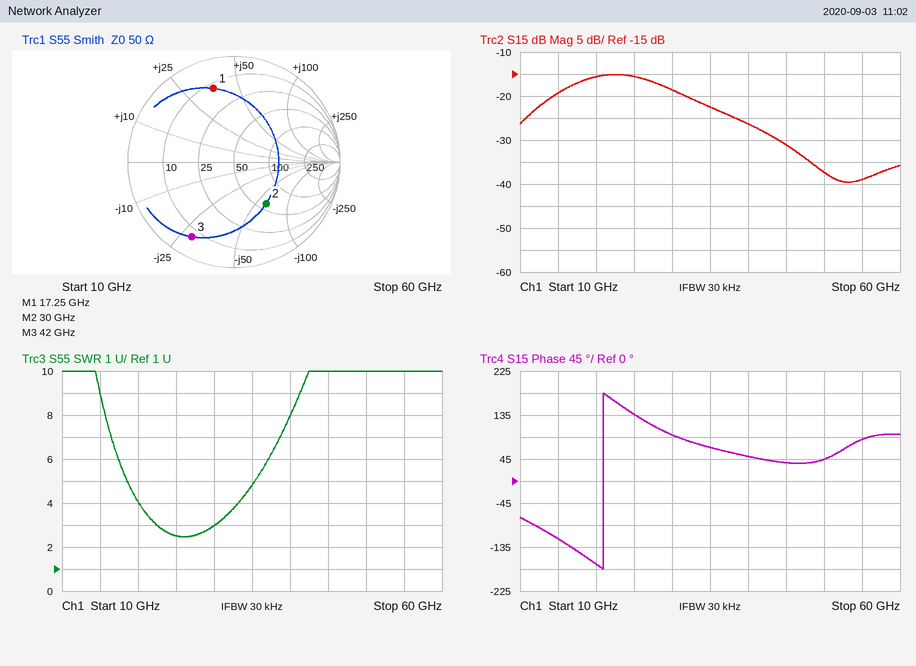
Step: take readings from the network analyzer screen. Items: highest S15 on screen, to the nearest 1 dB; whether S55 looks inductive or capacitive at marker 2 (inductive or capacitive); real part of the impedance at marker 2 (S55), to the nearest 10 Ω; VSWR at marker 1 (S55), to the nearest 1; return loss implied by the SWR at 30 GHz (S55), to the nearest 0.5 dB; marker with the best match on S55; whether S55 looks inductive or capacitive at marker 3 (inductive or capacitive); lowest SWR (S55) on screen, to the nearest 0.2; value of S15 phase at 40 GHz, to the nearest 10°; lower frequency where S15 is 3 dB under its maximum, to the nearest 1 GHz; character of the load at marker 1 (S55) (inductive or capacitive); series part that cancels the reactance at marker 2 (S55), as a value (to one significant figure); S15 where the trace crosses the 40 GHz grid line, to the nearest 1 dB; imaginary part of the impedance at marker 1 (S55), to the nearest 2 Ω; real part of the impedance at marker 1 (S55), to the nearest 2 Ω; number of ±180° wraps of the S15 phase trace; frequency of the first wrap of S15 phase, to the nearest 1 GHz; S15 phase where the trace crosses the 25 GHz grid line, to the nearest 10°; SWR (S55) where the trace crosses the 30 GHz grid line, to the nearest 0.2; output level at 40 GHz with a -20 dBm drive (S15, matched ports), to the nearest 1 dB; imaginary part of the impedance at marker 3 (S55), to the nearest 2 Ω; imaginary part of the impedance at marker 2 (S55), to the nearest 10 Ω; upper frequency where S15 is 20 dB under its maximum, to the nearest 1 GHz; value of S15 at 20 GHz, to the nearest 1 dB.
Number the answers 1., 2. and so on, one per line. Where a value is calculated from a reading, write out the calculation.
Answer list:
1. -15 dB
2. capacitive
3. 60 Ω
4. 6
5. −20 log10((3 − 1)/(3 + 1)) ≈ 6.0 dB
6. marker 2
7. capacitive
8. 2.4
9. 50°
10. 16 GHz
11. inductive
12. L = 60 Ω/(2π × 30 GHz) ≈ 318 pH, so 300 pH to one significant figure
13. -26 dB
14. +36 Ω
15. 12 Ω
16. 1
17. 21 GHz
18. 140°
19. 3.0
20. -20 dBm + (-26 dB) = -46 dBm
21. -28 Ω
22. -60 Ω
23. 48 GHz
24. -16 dB
